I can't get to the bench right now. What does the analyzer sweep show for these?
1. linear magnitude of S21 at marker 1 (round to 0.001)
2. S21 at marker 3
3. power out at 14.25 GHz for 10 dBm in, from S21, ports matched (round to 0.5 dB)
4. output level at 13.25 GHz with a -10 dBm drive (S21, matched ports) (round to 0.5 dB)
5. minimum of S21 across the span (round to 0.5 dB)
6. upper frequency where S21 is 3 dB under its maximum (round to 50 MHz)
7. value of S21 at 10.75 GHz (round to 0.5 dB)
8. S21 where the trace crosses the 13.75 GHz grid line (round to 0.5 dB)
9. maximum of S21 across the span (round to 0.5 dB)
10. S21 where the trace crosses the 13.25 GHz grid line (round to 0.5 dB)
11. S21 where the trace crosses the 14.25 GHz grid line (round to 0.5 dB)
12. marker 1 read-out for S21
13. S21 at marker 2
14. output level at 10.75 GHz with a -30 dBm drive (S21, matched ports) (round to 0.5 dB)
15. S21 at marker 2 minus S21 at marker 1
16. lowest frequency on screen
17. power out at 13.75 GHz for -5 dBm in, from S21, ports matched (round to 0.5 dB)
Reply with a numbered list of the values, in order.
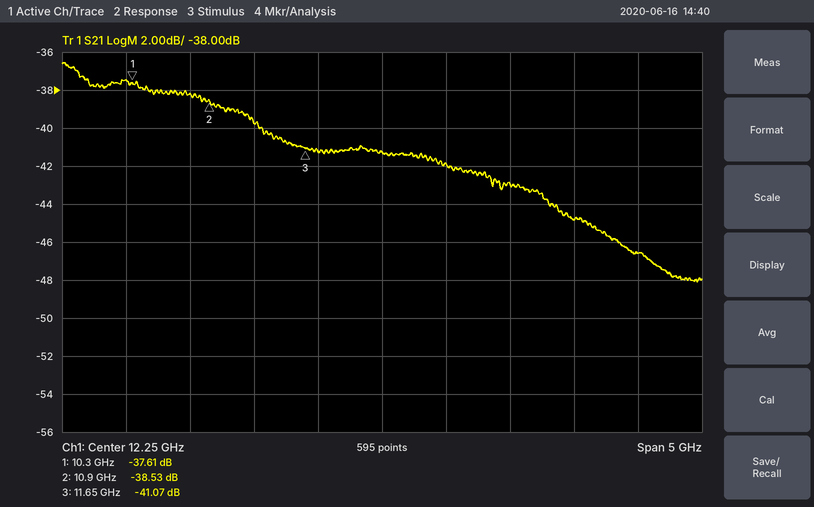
1. 0.013
2. -41.07 dB
3. -36.5 dBm
4. -53.0 dBm
5. -48.0 dB
6. 11.25 GHz
7. -38.0 dB
8. -45.0 dB
9. -36.5 dB
10. -43.0 dB
11. -46.5 dB
12. -37.61 dB
13. -38.53 dB
14. -68.0 dBm
15. -0.92 dB
16. 9.75 GHz
17. -50.0 dBm
